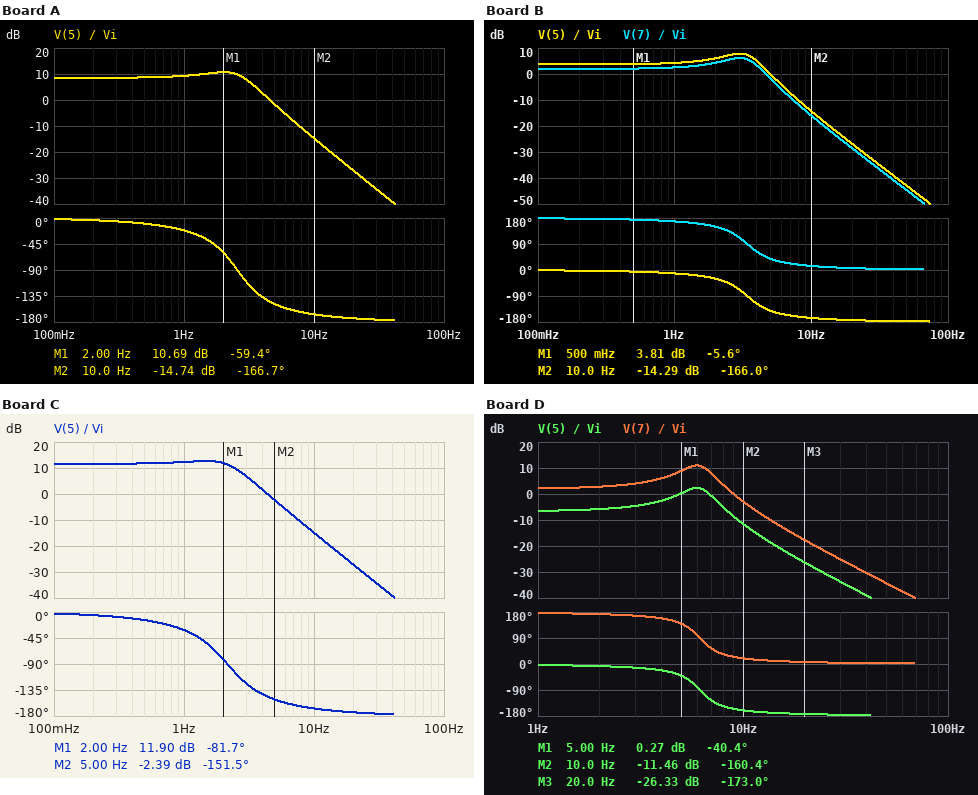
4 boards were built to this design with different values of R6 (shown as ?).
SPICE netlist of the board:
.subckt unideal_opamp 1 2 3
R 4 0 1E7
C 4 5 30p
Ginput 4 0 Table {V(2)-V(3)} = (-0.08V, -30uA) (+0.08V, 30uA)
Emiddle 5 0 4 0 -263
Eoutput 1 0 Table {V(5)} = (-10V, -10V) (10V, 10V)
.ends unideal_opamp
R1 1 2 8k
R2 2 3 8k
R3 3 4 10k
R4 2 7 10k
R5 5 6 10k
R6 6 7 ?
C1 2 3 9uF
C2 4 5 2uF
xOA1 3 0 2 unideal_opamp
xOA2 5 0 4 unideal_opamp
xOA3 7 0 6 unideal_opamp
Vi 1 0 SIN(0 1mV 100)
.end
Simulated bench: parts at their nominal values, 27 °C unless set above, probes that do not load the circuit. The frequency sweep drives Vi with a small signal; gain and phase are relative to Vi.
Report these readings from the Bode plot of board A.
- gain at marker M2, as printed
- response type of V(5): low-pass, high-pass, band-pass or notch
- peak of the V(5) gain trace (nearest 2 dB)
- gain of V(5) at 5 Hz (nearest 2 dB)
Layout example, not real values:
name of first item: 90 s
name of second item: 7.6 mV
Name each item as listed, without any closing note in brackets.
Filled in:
gain at marker M2, as printed: -14.74 dB
response type of V(5): low-pass, high-pass, band-pass or notch: low-pass
peak of the V(5) gain trace: 10 dB
gain of V(5) at 5 Hz: -2 dB
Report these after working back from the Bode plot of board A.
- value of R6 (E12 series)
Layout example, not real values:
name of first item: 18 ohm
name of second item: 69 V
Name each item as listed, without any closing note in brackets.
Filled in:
value of R6: 4.7 kΩ
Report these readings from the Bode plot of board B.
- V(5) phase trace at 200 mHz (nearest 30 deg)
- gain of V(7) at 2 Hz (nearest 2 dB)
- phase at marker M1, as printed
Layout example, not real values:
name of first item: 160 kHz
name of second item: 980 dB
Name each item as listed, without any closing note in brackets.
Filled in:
V(5) phase trace at 200 mHz: 0 deg
gain of V(7) at 2 Hz: 4 dB
phase at marker M1, as printed: -5.6 deg
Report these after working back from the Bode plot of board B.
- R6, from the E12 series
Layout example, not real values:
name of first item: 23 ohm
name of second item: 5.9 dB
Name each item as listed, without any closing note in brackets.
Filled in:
R6, from the E12 series: 8.2 kΩ
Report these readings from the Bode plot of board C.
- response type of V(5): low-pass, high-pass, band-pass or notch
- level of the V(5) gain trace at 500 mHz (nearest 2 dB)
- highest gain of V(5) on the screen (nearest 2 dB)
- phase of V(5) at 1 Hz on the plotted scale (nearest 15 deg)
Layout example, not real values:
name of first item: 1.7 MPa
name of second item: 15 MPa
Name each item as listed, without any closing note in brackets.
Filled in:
response type of V(5): low-pass, high-pass, band-pass or notch: low-pass
level of the V(5) gain trace at 500 mHz: 12 dB
highest gain of V(5) on the screen: 12 dB
phase of V(5) at 1 Hz on the plotted scale: -30 deg
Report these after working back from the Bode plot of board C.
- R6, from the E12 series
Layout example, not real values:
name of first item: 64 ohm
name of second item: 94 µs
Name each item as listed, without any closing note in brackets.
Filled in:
R6, from the E12 series: 3.3 kΩ
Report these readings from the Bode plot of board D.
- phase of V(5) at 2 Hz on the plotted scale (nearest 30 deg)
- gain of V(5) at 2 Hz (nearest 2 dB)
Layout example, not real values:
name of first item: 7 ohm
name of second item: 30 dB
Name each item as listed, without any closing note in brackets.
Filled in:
phase of V(5) at 2 Hz on the plotted scale: 0 deg
gain of V(5) at 2 Hz: -6 dB
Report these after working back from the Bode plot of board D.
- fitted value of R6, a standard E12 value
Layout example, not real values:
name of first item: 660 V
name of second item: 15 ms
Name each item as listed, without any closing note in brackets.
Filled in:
fitted value of R6, a standard E12 value: 27 kΩ
